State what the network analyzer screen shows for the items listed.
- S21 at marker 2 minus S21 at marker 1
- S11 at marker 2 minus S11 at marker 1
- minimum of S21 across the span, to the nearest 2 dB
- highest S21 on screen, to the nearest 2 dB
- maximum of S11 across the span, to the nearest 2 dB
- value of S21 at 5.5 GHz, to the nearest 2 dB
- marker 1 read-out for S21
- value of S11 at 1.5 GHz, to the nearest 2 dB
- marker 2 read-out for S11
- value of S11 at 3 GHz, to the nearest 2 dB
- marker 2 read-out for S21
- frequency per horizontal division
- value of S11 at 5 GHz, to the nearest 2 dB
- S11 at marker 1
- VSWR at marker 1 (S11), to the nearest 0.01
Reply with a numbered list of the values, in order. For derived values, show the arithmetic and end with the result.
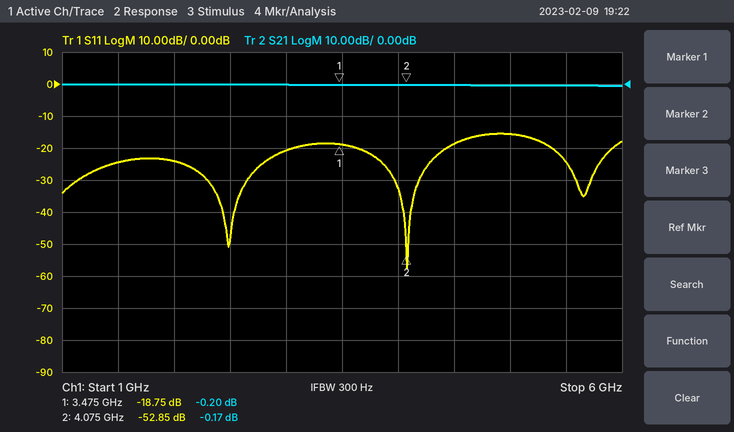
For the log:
1. -0.17 − (-0.2) = 0.03 dB
2. -52.85 − (-18.75) = -34.10 dB
3. 0 dB
4. 0 dB
5. -16 dB
6. 0 dB
7. -0.20 dB
8. -24 dB
9. -52.85 dB
10. -20 dB
11. -0.17 dB
12. 500 MHz
13. -16 dB
14. -18.75 dB
15. (1 + 0.1155)/(1 − 0.1155) ≈ 1.26
